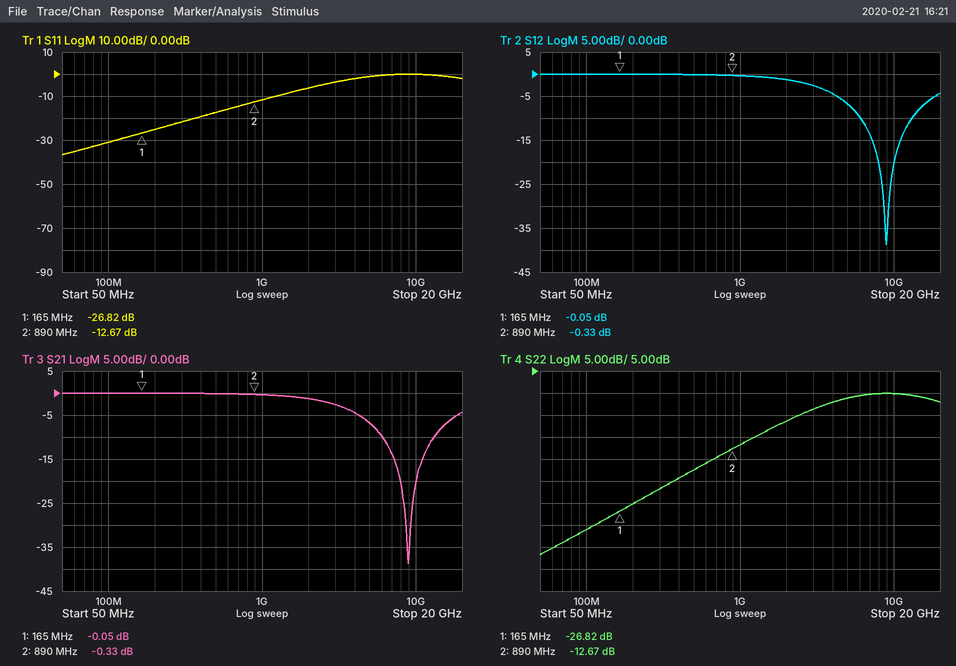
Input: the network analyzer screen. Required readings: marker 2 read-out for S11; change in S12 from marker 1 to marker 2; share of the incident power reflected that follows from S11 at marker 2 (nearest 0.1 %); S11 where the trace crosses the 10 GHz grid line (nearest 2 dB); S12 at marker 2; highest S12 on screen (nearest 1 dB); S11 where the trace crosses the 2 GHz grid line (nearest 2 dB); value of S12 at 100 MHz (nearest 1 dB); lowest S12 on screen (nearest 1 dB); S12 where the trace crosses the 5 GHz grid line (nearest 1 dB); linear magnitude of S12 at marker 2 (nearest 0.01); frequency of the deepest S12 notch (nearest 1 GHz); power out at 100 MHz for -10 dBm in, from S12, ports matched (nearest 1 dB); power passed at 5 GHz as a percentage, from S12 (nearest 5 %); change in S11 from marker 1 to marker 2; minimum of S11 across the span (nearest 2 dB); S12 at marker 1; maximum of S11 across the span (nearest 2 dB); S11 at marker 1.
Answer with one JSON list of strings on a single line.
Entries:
["-12.67 dB", "-0.28 dB", "5.4 %", "0 dB", "-0.33 dB", "0 dB", "-6 dB", "0 dB", "-39 dB", "-7 dB", "0.96", "9 GHz", "-10 dBm", "20 %", "14.15 dB", "-36 dB", "-0.05 dB", "0 dB", "-26.82 dB"]
